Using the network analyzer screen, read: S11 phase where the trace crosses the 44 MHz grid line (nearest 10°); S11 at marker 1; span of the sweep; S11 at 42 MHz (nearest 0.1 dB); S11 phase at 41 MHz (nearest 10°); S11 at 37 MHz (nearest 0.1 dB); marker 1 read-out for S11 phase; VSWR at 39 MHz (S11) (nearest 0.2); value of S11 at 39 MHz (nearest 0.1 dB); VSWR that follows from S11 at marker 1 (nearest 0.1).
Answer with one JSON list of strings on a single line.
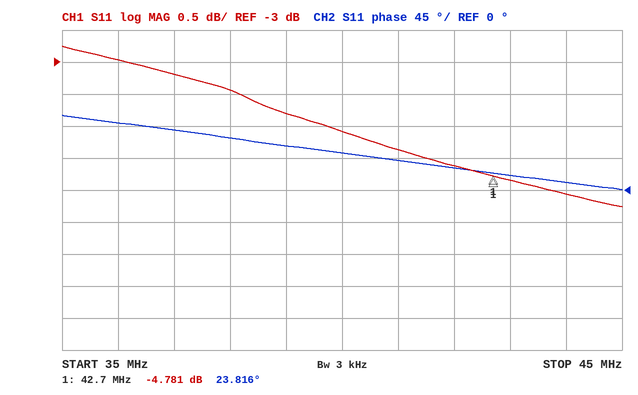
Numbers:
["10°", "-4.781 dB", "10 MHz", "-4.6 dB", "40°", "-3.2 dB", "23.816°", "4.6", "-3.8 dB", "3.7"]
